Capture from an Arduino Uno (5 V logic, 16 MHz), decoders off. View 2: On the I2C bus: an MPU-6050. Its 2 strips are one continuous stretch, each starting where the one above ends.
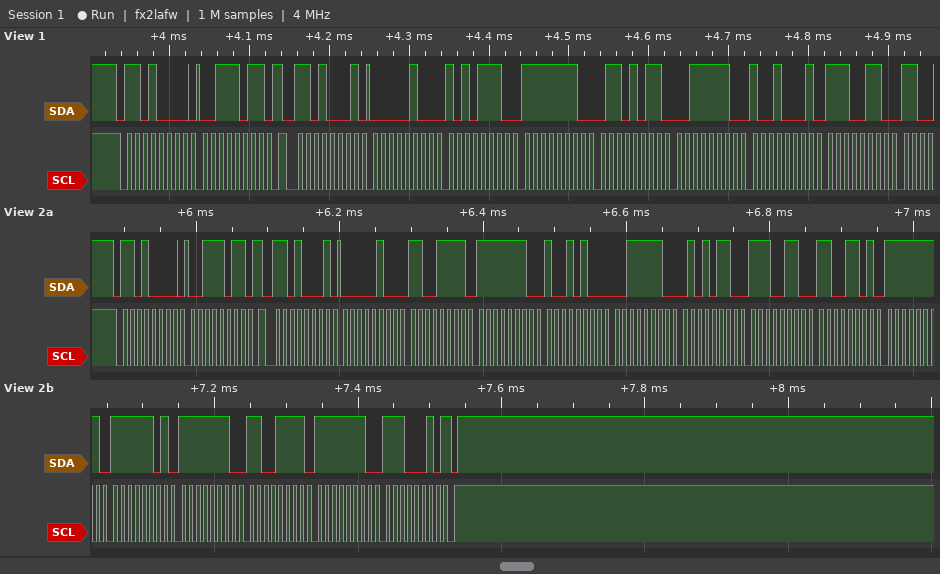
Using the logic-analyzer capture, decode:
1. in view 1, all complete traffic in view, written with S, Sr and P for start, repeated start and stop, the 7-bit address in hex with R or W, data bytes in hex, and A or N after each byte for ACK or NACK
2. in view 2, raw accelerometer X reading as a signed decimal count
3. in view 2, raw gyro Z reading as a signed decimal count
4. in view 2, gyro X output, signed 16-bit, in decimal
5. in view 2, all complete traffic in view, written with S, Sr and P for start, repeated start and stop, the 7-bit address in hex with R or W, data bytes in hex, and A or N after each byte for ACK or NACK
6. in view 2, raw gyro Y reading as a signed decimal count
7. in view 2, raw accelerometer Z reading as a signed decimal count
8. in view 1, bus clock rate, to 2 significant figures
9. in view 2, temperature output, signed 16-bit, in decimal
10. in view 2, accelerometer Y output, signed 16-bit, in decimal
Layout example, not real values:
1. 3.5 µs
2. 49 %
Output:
1. S 68W A 3B A Sr 68R A 04 A AE A FE A 6B A 3E A 91 A E6 A
2. 1231
3. -286
4. -3
5. S 68W A 3B A Sr 68R A 04 A CF A FE A 94 A 3E A 56 A E6 A CD A FF A FD A FE A CF A FE A E2 N P
6. -305
7. 15958
8. 100 kHz
9. -6451
10. -364
